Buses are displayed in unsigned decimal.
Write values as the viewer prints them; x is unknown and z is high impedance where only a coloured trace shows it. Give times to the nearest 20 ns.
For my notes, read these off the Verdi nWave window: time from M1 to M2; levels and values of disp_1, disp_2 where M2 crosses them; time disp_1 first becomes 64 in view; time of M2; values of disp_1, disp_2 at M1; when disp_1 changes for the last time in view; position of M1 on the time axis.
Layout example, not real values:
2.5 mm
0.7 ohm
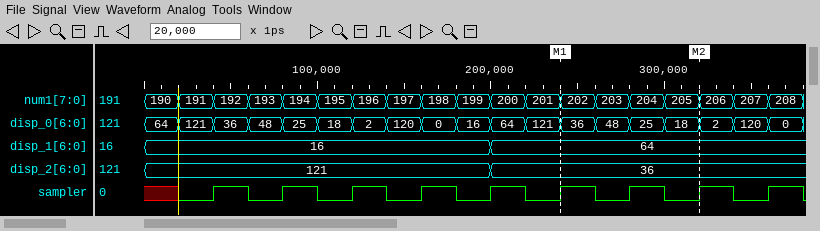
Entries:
80 ns
disp_1=64, disp_2=36
200 ns
320 ns
disp_1=64, disp_2=36
200 ns
240 ns
